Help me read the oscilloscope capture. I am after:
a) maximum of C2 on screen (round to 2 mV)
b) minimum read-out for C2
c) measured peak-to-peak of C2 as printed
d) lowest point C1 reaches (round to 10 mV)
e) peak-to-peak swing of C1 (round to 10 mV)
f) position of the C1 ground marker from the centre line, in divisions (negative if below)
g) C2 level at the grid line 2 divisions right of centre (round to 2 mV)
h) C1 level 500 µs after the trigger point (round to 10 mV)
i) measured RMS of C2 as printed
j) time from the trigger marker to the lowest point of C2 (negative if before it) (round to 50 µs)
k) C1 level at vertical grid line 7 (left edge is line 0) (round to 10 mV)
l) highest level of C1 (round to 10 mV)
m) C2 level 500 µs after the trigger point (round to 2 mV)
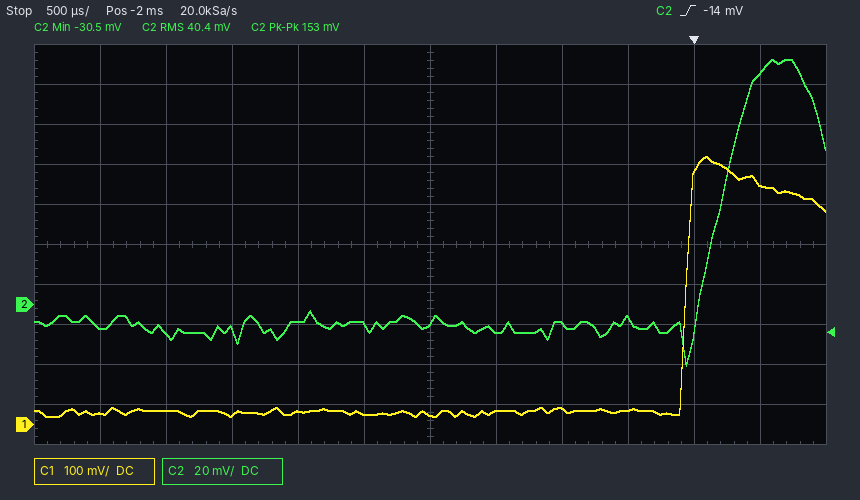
122 mV
-30.5 mV
153 mV
20 mV
650 mV
-4.5 div
-10 mV
600 mV
40.4 mV
-50 µs
30 mV
670 mV
116 mV
